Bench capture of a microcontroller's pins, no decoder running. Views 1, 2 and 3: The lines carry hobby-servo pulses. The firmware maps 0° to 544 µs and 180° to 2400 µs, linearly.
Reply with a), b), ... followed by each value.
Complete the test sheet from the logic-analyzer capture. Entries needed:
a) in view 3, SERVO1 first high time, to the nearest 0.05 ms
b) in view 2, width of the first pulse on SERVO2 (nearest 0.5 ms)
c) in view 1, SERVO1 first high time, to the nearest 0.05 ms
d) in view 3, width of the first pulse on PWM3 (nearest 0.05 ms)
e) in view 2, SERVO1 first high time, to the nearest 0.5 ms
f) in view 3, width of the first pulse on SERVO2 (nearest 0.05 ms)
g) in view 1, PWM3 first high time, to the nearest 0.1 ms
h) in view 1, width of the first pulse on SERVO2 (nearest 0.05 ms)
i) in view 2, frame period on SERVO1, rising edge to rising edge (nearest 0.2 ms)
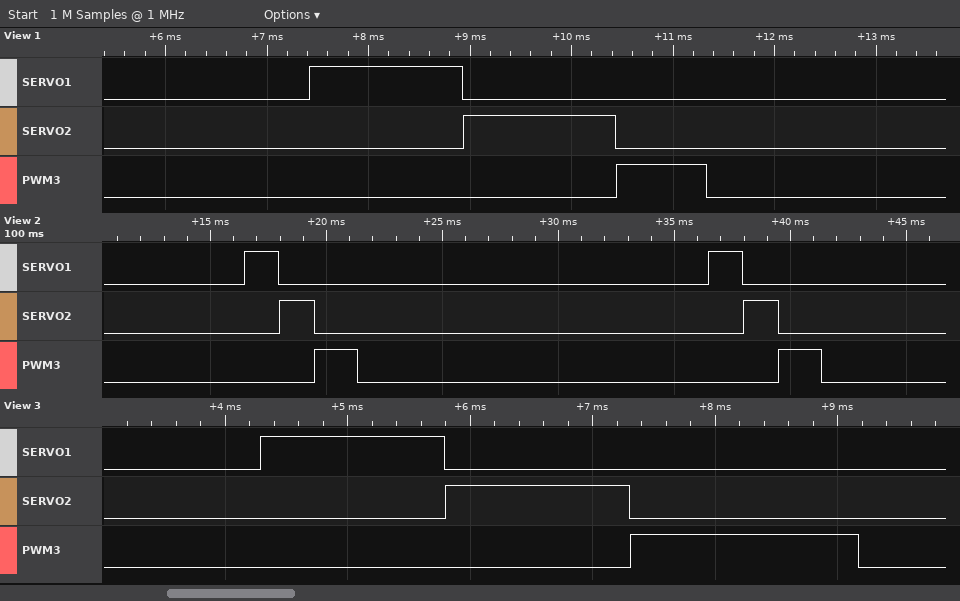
a) 1.50 ms
b) 1.5 ms
c) 1.50 ms
d) 1.85 ms
e) 1.5 ms
f) 1.50 ms
g) 0.9 ms
h) 1.50 ms
i) 20.0 ms
